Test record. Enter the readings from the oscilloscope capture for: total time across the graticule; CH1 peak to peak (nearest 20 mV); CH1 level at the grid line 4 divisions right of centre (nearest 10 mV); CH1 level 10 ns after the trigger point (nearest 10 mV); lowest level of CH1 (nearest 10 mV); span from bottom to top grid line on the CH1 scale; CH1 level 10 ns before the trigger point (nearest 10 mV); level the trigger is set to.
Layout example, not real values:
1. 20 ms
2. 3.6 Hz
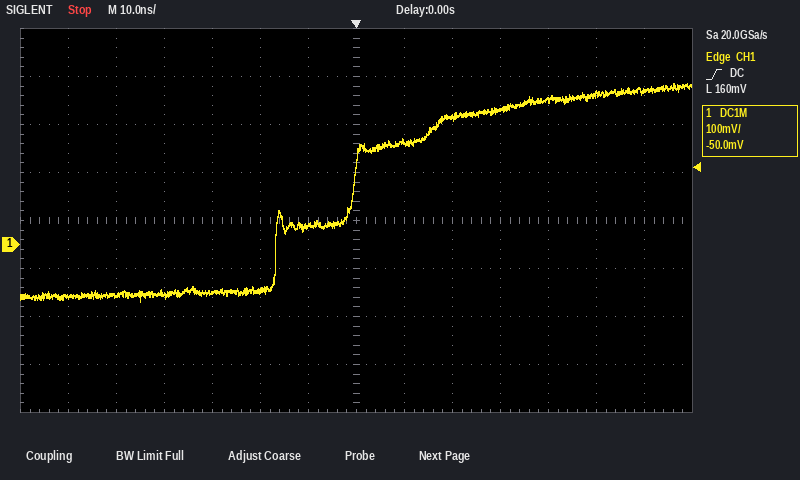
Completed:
1. 140 ns
2. 460 mV
3. 300 mV
4. 210 mV
5. -120 mV
6. 800 mV
7. 40 mV
8. 160 mV
